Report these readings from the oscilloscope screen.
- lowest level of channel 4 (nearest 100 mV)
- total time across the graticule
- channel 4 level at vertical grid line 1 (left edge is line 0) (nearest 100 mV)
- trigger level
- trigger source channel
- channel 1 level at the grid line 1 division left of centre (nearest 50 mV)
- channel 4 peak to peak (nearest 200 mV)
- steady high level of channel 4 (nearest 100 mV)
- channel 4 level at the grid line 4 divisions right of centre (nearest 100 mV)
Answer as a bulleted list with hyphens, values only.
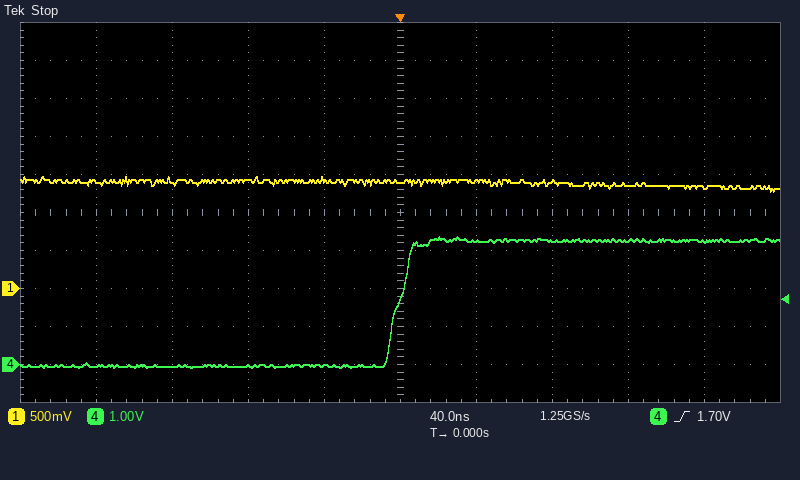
- -100 mV
- 400 ns
- 0.0 V
- 1.70 V
- channel 4
- 1.45 V
- 3.4 V
- 3.3 V
- 3.2 V
